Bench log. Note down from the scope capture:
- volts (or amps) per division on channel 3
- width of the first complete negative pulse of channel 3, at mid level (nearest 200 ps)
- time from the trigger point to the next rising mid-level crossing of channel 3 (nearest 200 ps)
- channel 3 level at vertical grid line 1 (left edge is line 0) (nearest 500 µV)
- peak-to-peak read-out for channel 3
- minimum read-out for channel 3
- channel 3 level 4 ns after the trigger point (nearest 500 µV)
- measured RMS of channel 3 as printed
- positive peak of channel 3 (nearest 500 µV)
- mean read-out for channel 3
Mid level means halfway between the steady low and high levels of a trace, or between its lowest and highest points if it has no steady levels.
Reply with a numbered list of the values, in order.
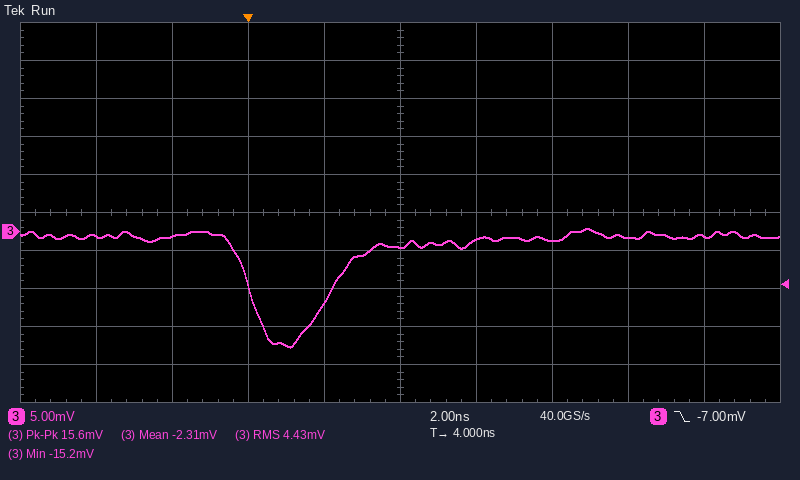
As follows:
1. 5 mV
2. 2.2 ns
3. 2.2 ns
4. -500 µV
5. 15.6 mV
6. -15.2 mV
7. -2.0 mV
8. 4.43 mV
9. 500 µV
10. -2.31 mV
